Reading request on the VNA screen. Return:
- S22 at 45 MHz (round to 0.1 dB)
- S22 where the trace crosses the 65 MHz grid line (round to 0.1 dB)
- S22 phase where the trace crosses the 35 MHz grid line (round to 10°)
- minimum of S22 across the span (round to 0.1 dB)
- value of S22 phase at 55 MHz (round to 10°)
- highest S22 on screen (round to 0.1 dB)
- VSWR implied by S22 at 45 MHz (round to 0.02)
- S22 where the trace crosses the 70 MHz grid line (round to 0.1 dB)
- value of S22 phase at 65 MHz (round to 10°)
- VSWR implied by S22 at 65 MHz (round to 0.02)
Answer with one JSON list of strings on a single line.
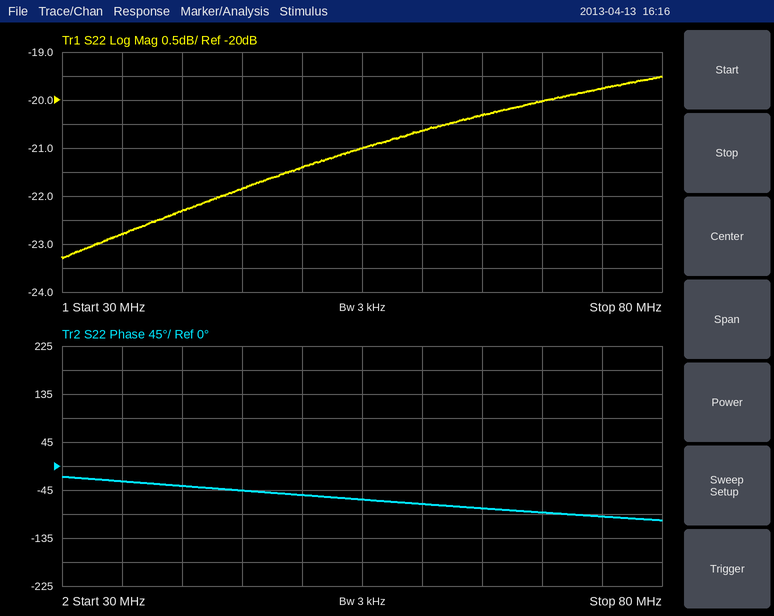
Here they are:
["-21.8 dB", "-20.3 dB", "-30°", "-23.3 dB", "-60°", "-19.5 dB", "1.18", "-20.0 dB", "-80°", "1.22"]
